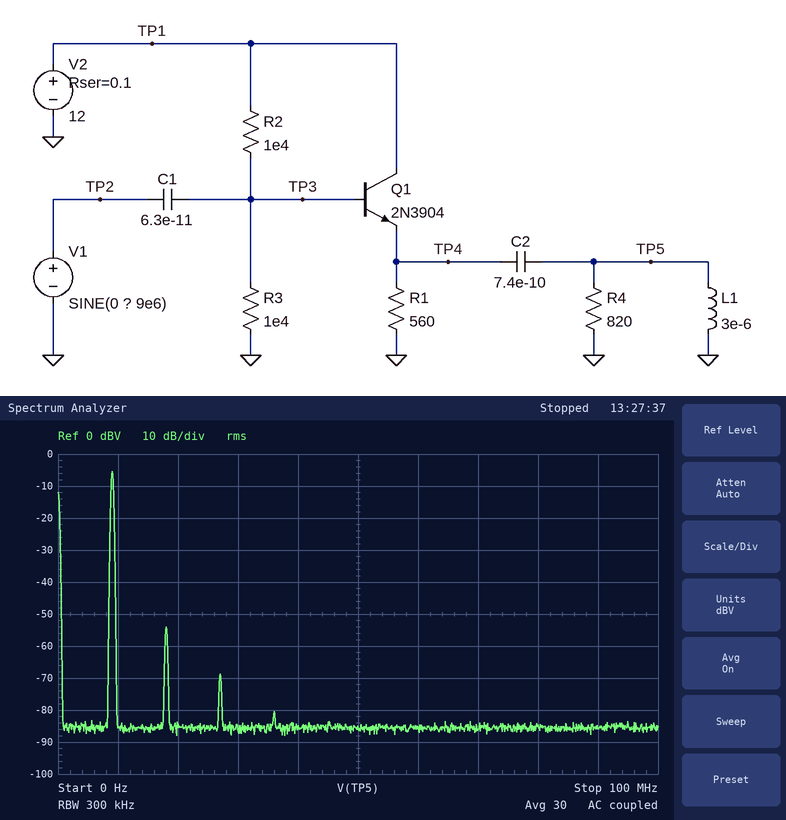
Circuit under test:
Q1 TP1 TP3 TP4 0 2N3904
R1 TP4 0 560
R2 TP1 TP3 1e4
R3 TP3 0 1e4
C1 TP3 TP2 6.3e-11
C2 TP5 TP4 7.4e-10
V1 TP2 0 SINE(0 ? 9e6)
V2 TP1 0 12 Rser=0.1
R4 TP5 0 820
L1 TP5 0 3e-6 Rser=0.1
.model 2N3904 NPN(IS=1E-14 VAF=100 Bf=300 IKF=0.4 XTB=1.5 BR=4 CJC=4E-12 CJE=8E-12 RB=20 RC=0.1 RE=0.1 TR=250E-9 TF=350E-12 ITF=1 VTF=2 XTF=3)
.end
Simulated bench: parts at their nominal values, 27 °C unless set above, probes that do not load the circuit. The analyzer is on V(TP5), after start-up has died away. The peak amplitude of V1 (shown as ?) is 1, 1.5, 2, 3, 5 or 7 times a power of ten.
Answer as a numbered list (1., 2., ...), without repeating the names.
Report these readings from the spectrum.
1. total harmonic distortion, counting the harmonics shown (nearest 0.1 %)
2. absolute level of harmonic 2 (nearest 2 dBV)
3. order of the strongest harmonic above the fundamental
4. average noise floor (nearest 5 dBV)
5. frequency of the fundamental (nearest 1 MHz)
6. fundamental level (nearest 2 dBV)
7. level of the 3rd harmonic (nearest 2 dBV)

1. 0.4 %
2. -54 dBV
3. 2
4. -85 dBV
5. 9 MHz
6. -6 dBV
7. -68 dBV
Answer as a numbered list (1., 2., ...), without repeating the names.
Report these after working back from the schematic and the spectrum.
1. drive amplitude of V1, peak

1. 700 mV
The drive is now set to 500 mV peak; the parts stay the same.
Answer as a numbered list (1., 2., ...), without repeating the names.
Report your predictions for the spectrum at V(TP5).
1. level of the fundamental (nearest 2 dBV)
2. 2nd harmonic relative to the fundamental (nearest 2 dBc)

1. -8 dBV
2. -52 dBc
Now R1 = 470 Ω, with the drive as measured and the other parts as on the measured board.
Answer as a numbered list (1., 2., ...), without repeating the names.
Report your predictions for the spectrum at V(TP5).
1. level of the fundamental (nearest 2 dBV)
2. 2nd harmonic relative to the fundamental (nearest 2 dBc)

1. -6 dBV
2. -52 dBc
